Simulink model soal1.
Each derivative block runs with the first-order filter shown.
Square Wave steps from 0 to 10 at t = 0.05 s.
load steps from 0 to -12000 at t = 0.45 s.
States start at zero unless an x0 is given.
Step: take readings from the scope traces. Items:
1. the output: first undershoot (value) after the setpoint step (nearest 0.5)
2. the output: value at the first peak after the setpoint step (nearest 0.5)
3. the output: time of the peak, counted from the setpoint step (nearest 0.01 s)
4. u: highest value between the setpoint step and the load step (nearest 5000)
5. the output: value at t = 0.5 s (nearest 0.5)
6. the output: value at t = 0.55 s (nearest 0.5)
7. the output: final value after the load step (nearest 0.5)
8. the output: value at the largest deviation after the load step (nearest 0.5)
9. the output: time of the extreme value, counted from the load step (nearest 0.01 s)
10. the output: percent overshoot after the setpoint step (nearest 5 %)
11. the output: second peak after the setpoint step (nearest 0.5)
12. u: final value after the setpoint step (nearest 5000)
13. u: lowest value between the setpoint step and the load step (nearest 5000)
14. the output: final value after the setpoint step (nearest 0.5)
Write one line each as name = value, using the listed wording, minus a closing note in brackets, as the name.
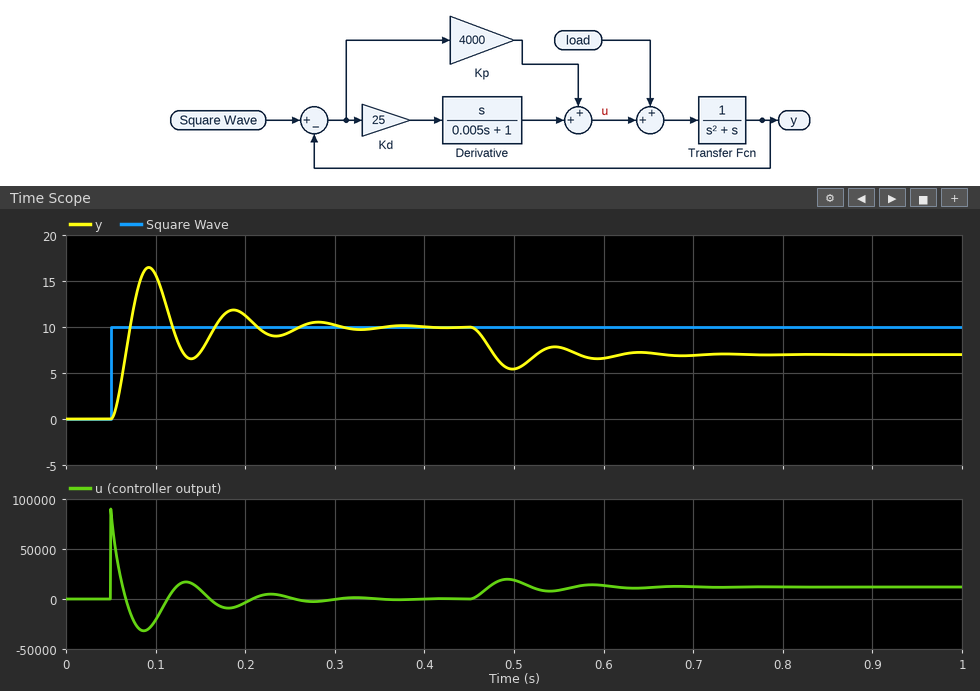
the output: first undershoot (value) after the setpoint step = 6.5
the output: value at the first peak after the setpoint step = 16.5
the output: time of the peak, counted from the setpoint step = 0.04 s
u: highest value between the setpoint step and the load step = 90000
the output: value at t = 0.5 s = 5.5
the output: value at t = 0.55 s = 8.0
the output: final value after the load step = 7.0
the output: value at the largest deviation after the load step = 5.5
the output: time of the extreme value, counted from the load step = 0.05 s
the output: percent overshoot after the setpoint step = 65 %
the output: second peak after the setpoint step = 12.0
u: final value after the setpoint step = 0
u: lowest value between the setpoint step and the load step = -30000
the output: final value after the setpoint step = 10.0
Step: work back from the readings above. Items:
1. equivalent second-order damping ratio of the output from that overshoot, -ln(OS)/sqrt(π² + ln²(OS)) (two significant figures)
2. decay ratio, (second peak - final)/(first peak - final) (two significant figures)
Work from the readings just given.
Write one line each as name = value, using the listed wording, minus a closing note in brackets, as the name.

equivalent second-order damping ratio of the output from that overshoot, -ln(OS)/sqrt(π² + ln²(OS)) = 0.14
decay ratio, (second peak - final)/(first peak - final) = 0.31
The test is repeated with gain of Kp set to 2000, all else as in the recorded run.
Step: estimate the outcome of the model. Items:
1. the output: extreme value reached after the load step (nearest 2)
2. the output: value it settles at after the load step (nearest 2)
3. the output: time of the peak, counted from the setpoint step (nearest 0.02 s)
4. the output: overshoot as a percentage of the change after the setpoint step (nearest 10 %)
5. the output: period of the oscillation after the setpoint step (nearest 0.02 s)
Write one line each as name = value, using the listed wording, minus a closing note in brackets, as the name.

the output: extreme value reached after the load step = 2
the output: value it settles at after the load step = 4
the output: time of the peak, counted from the setpoint step = 0.06 s
the output: overshoot as a percentage of the change after the setpoint step = 50 %
the output: period of the oscillation after the setpoint step = 0.14 s
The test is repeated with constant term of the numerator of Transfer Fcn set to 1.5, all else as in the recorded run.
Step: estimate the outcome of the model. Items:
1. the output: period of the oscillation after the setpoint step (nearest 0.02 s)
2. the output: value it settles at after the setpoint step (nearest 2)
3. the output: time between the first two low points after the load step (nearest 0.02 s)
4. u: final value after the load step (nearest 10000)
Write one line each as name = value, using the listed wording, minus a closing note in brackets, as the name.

the output: period of the oscillation after the setpoint step = 0.08 s
the output: value it settles at after the setpoint step = 10
the output: time between the first two low points after the load step = 0.08 s
u: final value after the load step = 10000
